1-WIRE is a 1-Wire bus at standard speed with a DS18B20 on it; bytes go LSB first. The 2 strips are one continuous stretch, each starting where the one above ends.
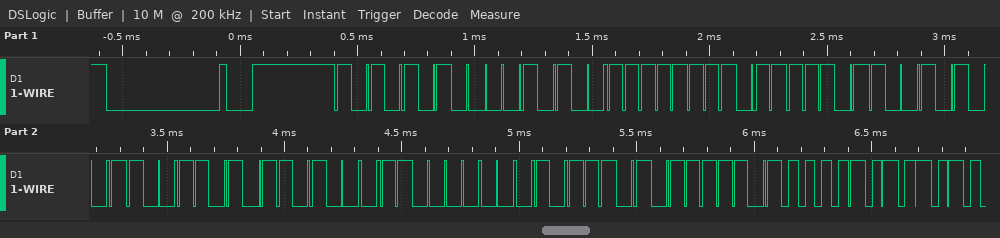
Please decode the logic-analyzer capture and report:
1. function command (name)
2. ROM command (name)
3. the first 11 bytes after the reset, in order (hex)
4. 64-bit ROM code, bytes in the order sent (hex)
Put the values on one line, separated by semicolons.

Read Scratchpad; Match ROM; 55 28 FF BE 29 B3 16 03 BA BE 50; 28 FF BE 29 B3 16 03 BA
